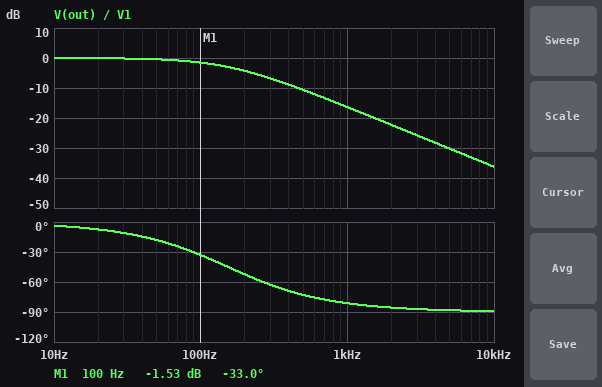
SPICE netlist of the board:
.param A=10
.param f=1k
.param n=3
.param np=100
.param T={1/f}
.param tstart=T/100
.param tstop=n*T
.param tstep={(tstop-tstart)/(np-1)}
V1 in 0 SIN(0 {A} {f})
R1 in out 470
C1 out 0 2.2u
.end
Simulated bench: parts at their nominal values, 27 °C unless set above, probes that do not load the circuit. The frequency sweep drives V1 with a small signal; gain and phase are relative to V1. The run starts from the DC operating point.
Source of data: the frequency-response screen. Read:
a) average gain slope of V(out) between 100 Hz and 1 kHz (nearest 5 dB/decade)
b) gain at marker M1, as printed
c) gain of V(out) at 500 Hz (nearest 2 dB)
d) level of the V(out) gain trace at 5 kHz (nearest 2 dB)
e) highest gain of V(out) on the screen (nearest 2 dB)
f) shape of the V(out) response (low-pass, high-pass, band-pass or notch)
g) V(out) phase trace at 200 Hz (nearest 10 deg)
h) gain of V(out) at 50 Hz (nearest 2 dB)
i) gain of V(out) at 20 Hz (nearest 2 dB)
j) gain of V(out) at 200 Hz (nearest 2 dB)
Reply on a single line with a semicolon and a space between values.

-15 dB/decade; -1.53 dB; -10 dB; -30 dB; 0 dB; low-pass; -50 deg; 0 dB; 0 dB; -4 dB
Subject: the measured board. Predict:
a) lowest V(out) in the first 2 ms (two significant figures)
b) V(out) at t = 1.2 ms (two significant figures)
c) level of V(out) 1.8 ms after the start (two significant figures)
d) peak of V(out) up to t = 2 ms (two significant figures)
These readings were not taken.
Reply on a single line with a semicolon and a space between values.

-1.3 V; 230 mV; -420 mV; 2.5 V
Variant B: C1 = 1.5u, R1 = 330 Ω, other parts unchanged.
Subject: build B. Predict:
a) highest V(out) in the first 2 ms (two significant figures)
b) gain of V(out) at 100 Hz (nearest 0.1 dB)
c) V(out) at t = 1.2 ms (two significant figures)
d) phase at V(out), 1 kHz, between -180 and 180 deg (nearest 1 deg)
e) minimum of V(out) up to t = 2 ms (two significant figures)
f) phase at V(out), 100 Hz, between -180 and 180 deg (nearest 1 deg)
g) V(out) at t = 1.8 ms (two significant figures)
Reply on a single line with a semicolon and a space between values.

4.3 V; -0.4 dB; 250 mV; -72 deg; -3.0 V; -17 deg; -1.7 V
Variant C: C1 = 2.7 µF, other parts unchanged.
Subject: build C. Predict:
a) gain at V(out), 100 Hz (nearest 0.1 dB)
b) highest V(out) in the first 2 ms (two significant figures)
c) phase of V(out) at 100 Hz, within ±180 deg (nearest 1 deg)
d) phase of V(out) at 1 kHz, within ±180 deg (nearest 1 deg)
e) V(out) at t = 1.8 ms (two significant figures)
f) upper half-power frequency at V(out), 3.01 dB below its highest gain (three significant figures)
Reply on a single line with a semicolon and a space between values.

-2.1 dB; 2.1 V; -39 deg; -83 deg; -230 mV; 125 Hz
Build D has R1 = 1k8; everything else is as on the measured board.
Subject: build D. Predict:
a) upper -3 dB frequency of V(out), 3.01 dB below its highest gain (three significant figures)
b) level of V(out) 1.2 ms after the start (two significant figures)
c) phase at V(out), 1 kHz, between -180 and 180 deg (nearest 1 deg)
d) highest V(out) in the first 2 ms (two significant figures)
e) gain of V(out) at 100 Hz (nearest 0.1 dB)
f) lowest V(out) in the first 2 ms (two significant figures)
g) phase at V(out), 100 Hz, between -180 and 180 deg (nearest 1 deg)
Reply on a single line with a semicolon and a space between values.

40.2 Hz; 190 mV; -88 deg; 760 mV; -8.6 dB; -160 mV; -68 deg
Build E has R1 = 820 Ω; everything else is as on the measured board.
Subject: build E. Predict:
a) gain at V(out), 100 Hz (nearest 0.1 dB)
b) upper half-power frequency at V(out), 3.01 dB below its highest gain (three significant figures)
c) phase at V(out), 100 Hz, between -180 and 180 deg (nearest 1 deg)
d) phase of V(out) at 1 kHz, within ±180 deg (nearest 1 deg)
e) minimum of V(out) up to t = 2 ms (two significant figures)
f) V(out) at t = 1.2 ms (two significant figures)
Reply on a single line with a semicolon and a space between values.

-3.6 dB; 88.2 Hz; -49 deg; -85 deg; -590 mV; 250 mV
